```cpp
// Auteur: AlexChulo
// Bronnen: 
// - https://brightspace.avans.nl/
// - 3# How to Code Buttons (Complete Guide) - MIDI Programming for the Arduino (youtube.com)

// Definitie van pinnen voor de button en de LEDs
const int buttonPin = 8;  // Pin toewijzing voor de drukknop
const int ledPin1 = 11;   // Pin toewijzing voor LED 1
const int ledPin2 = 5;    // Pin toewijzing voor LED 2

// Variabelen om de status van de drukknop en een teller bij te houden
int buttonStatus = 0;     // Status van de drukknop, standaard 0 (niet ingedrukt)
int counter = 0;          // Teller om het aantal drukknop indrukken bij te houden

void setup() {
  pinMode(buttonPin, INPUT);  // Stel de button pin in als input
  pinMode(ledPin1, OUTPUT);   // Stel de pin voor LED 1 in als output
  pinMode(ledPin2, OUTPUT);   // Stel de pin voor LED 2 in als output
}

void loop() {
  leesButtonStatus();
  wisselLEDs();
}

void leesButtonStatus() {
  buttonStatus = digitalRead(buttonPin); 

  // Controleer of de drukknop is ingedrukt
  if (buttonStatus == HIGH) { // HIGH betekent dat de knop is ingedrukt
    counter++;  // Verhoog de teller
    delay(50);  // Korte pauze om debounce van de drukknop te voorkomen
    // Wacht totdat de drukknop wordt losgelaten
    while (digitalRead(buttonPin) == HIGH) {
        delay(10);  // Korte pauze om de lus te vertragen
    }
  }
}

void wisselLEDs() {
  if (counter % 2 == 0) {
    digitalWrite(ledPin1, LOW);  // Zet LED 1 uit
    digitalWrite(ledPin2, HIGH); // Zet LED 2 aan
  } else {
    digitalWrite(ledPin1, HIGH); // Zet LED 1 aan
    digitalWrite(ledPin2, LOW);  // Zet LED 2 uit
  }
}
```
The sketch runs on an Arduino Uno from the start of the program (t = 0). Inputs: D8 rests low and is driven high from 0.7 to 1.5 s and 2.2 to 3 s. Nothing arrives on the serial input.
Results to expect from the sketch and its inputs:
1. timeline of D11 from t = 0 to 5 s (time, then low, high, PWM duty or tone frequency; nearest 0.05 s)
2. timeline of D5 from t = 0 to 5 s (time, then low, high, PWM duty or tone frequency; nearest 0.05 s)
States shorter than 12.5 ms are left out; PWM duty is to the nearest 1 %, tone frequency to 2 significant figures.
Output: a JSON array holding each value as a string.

["0 s low; 1.5 s high; 3 s low", "0 s high; 1.5 s low; 3 s high"]
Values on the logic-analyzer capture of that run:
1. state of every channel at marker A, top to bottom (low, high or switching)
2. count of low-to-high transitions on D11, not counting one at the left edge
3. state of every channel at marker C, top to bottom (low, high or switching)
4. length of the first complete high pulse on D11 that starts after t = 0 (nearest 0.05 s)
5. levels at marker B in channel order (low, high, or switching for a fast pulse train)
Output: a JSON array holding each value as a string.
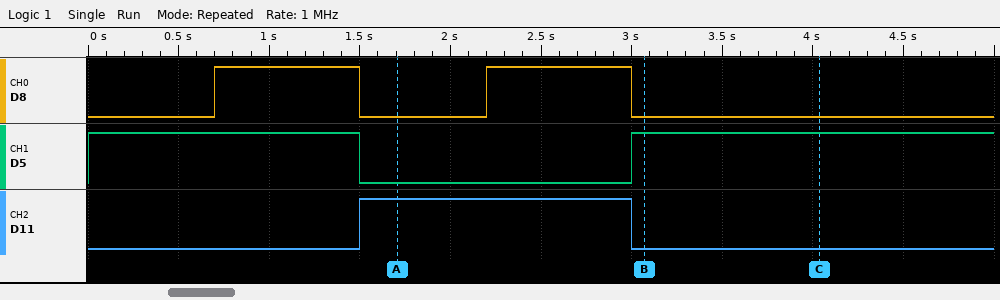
["D8 low, D5 low, D11 high", "1", "D8 low, D5 high, D11 low", "1.50 s", "D8 low, D5 high, D11 low"]
